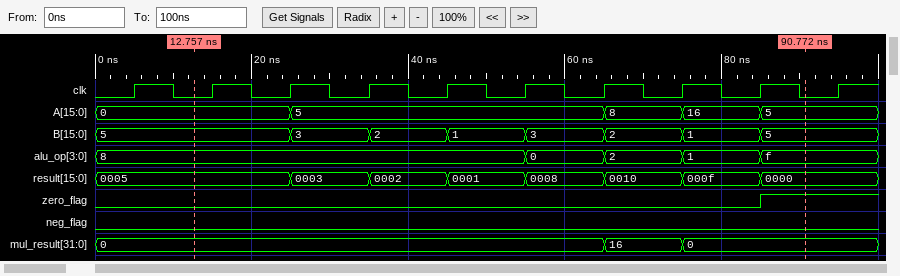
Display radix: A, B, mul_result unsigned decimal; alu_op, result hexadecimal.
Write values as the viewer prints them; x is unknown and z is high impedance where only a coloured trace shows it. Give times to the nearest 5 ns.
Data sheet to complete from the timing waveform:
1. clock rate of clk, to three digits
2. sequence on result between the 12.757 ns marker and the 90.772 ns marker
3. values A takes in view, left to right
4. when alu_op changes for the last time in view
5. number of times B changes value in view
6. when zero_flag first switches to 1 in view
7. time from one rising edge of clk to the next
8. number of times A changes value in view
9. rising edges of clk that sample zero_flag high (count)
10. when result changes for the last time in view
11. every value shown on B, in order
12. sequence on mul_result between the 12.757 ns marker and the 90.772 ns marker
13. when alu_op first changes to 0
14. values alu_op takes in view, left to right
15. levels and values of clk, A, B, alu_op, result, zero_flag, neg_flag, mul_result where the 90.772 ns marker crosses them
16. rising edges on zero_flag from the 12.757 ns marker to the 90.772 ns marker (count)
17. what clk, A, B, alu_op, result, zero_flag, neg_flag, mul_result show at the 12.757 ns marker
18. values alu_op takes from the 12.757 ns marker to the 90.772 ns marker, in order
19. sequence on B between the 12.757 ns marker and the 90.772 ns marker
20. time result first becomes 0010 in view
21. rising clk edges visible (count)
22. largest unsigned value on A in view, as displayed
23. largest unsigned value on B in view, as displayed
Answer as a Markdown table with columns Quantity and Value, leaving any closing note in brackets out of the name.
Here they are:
| Quantity | Value |
|---|---|
| clock rate of clk, to three digits | 100 MHz |
| sequence on result between the 12.757 ns marker and the 90.772 ns marker | 0005, 0003, 0002, 0001, 0008, 0010, 000f, 0000 |
| values A takes in view, left to right | 0, 5, 8, 16, 5 |
| when alu_op changes for the last time in view | 85 ns |
| number of times B changes value in view | 7 |
| when zero_flag first switches to 1 in view | 85 ns |
| time from one rising edge of clk to the next | 10 ns |
| number of times A changes value in view | 4 |
| rising edges of clk that sample zero_flag high | 1 |
| when result changes for the last time in view | 85 ns |
| every value shown on B, in order | 5, 3, 2, 1, 3, 2, 1, 5 |
| sequence on mul_result between the 12.757 ns marker and the 90.772 ns marker | 0, 16, 0 |
| when alu_op first changes to 0 | 55 ns |
| values alu_op takes in view, left to right | 8, 0, 2, 1, f |
| levels and values of clk, A, B, alu_op, result, zero_flag, neg_flag, mul_result where the 90.772 ns marker crosses them | clk=0, A=5, B=5, alu_op=f, result=0000, zero_flag=1, neg_flag=0, mul_result=0 |
| rising edges on zero_flag from the 12.757 ns marker to the 90.772 ns marker | 1 |
| what clk, A, B, alu_op, result, zero_flag, neg_flag, mul_result show at the 12.757 ns marker | clk=0, A=0, B=5, alu_op=8, result=0005, zero_flag=0, neg_flag=0, mul_result=0 |
| values alu_op takes from the 12.757 ns marker to the 90.772 ns marker, in order | 8, 0, 2, 1, f |
| sequence on B between the 12.757 ns marker and the 90.772 ns marker | 5, 3, 2, 1, 3, 2, 1, 5 |
| time result first becomes 0010 in view | 65 ns |
| rising clk edges visible | 10 |
| largest unsigned value on A in view, as displayed | 16 |
| largest unsigned value on B in view, as displayed | 5 |
